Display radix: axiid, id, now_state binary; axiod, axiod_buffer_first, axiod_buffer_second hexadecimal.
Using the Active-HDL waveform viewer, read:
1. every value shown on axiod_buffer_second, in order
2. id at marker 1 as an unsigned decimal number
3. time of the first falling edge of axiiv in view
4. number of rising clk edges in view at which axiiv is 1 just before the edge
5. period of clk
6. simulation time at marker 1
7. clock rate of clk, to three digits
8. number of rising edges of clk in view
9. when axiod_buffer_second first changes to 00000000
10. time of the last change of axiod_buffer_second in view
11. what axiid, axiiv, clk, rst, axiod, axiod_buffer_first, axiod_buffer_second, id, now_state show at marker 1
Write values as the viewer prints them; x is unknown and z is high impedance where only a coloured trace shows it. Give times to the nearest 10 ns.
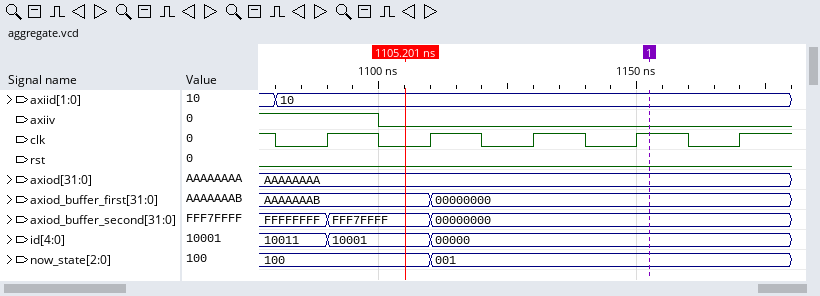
FFFFFFFF, FFF7FFFF, 00000000
0
1100 ns
1
20 ns
1150 ns
50.0 MHz
5
1110 ns
1110 ns
axiid=10, axiiv=0, clk=1, rst=0, axiod=AAAAAAAA, axiod_buffer_first=00000000, axiod_buffer_second=00000000, id=00000, now_state=001
